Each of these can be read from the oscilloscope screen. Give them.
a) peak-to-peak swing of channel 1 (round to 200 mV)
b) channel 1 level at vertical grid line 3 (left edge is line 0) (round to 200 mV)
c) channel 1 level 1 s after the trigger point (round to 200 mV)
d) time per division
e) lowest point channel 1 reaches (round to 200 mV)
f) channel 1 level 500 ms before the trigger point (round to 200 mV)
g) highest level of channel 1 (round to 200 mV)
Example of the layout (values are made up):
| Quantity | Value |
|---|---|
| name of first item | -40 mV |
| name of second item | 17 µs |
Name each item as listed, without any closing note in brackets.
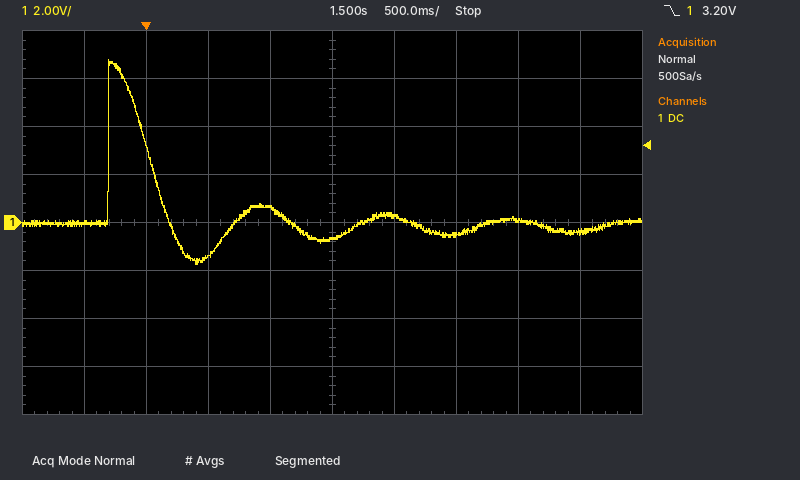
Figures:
| Quantity | Value |
|---|---|
| peak-to-peak swing of channel 1 | 8.6 V |
| channel 1 level at vertical grid line 3 (left edge is line 0) | -1.4 V |
| channel 1 level 1 s after the trigger point | 600 mV |
| time per division | 500 ms |
| lowest point channel 1 reaches | -1.8 V |
| channel 1 level 500 ms before the trigger point | 0.0 V |
| highest level of channel 1 | 6.8 V |
